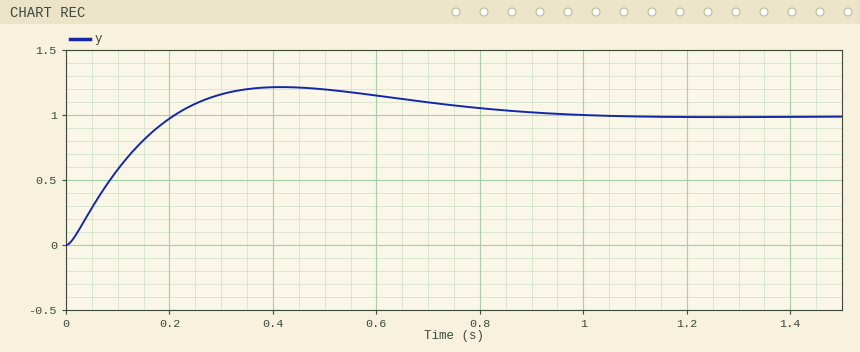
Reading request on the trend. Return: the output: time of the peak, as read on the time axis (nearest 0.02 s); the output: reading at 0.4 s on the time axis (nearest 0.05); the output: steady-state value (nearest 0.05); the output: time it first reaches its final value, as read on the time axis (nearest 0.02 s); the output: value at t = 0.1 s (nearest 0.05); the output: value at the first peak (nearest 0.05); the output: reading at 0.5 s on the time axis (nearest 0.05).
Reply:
0.42 s
1.20
1.00
0.20 s
0.60
1.20
1.20
